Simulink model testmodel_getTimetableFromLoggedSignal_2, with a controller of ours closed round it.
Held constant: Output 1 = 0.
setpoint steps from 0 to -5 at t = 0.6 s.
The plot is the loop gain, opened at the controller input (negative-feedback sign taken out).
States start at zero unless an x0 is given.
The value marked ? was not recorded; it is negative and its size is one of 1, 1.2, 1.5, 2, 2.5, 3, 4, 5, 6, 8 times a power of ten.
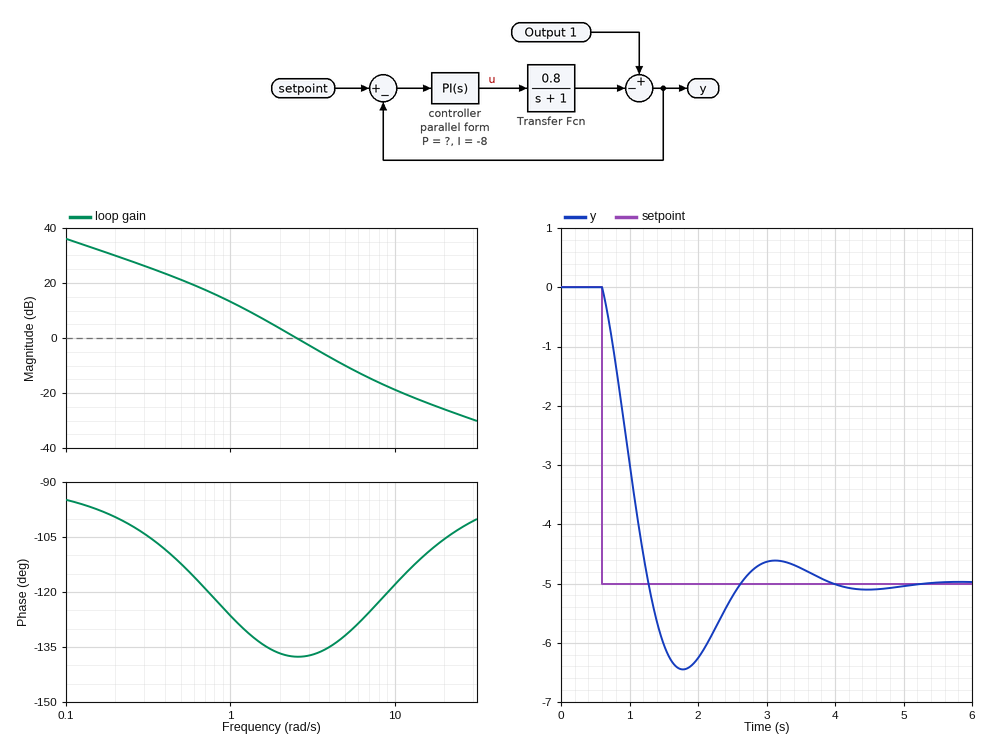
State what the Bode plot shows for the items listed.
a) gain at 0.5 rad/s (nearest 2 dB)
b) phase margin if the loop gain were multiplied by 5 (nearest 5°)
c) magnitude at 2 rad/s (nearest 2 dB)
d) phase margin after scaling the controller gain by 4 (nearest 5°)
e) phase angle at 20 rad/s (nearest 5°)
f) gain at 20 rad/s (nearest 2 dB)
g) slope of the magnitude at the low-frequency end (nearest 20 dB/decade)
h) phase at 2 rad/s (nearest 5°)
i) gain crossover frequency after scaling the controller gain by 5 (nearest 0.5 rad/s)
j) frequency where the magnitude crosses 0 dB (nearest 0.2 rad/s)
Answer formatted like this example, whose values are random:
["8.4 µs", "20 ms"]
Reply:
["22 dB", "55°", "4 dB", "50°", "-105°", "-26 dB", "-20 dB/decade", "-135°", "6.5 rad/s", "2.6 rad/s"]
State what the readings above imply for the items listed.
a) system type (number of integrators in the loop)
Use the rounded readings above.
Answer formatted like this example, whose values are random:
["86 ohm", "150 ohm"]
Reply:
["1"]
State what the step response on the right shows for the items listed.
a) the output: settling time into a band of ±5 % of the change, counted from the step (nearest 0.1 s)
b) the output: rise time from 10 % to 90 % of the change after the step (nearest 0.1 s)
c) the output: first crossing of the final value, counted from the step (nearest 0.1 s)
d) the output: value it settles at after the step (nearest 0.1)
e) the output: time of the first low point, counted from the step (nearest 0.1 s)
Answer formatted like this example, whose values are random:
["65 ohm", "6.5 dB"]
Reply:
["2.9 s", "0.5 s", "0.7 s", "-5.0", "1.2 s"]
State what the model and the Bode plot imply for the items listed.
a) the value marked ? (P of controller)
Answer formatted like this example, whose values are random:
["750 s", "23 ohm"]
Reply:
["-1.2"]
